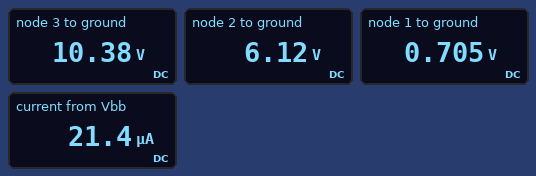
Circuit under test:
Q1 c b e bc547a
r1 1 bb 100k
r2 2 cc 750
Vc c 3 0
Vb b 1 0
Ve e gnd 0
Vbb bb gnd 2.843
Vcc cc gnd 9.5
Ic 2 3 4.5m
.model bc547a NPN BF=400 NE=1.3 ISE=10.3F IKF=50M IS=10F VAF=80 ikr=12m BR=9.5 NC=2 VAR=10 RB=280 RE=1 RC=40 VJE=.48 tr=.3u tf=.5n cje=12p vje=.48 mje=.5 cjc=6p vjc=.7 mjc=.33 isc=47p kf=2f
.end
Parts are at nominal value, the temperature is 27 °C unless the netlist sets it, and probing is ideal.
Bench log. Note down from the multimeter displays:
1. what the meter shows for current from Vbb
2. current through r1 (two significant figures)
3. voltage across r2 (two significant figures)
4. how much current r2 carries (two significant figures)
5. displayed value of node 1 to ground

21.4 µA
21 µA
3.4 V
4.5 mA
0.705 V
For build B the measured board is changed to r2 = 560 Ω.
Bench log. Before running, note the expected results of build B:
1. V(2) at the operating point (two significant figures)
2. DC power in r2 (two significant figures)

7.0 V
11 mW
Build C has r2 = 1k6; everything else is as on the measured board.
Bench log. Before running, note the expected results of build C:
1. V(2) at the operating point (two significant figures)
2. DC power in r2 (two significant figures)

2.3 V
32 mW
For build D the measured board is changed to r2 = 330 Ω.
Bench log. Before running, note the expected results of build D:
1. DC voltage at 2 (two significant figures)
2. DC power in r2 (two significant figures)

8.0 V
6.7 mW
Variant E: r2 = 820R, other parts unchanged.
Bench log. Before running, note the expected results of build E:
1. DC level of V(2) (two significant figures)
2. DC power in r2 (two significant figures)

5.8 V
17 mW
